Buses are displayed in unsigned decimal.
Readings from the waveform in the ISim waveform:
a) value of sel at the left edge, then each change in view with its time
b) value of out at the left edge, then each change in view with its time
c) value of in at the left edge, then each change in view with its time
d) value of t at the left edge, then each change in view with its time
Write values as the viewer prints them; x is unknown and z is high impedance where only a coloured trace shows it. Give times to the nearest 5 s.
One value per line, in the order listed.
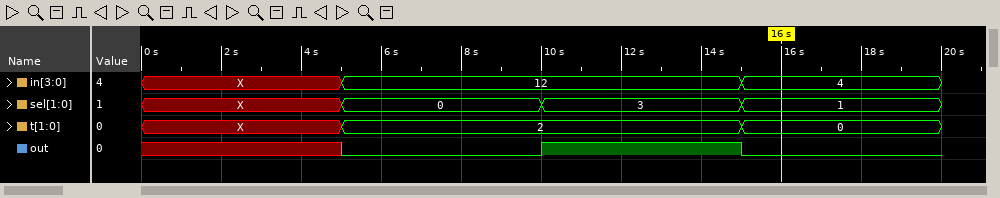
X, 0 at 5 s, 3 at 10 s, 1 at 15 s
x, 0 at 5 s, 1 at 10 s, 0 at 15 s
X, 12 at 5 s, 4 at 15 s
X, 2 at 5 s, 0 at 15 s
